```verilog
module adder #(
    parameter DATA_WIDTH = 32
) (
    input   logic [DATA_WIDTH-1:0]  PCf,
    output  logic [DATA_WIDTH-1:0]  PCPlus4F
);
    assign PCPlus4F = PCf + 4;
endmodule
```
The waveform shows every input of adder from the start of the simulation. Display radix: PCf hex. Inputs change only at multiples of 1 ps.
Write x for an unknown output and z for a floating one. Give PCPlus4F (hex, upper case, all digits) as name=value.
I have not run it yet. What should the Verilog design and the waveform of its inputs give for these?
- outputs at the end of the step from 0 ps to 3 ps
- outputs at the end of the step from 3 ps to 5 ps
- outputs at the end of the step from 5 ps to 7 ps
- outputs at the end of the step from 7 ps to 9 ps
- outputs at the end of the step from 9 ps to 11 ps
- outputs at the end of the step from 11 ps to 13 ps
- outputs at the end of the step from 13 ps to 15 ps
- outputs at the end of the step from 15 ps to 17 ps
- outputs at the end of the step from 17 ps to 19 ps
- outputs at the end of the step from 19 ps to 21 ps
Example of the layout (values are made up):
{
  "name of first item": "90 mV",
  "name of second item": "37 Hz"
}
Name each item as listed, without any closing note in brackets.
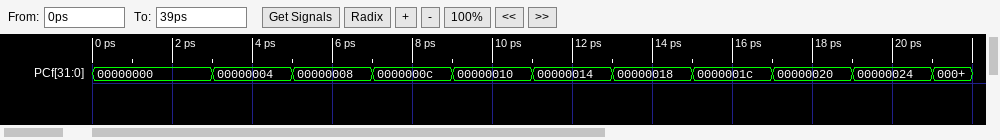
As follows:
{
  "outputs at the end of the step from 0 ps to 3 ps": "PCPlus4F=00000004",
  "outputs at the end of the step from 3 ps to 5 ps": "PCPlus4F=00000008",
  "outputs at the end of the step from 5 ps to 7 ps": "PCPlus4F=0000000C",
  "outputs at the end of the step from 7 ps to 9 ps": "PCPlus4F=00000010",
  "outputs at the end of the step from 9 ps to 11 ps": "PCPlus4F=00000014",
  "outputs at the end of the step from 11 ps to 13 ps": "PCPlus4F=00000018",
  "outputs at the end of the step from 13 ps to 15 ps": "PCPlus4F=0000001C",
  "outputs at the end of the step from 15 ps to 17 ps": "PCPlus4F=00000020",
  "outputs at the end of the step from 17 ps to 19 ps": "PCPlus4F=00000024",
  "outputs at the end of the step from 19 ps to 21 ps": "PCPlus4F=00000028"
}
